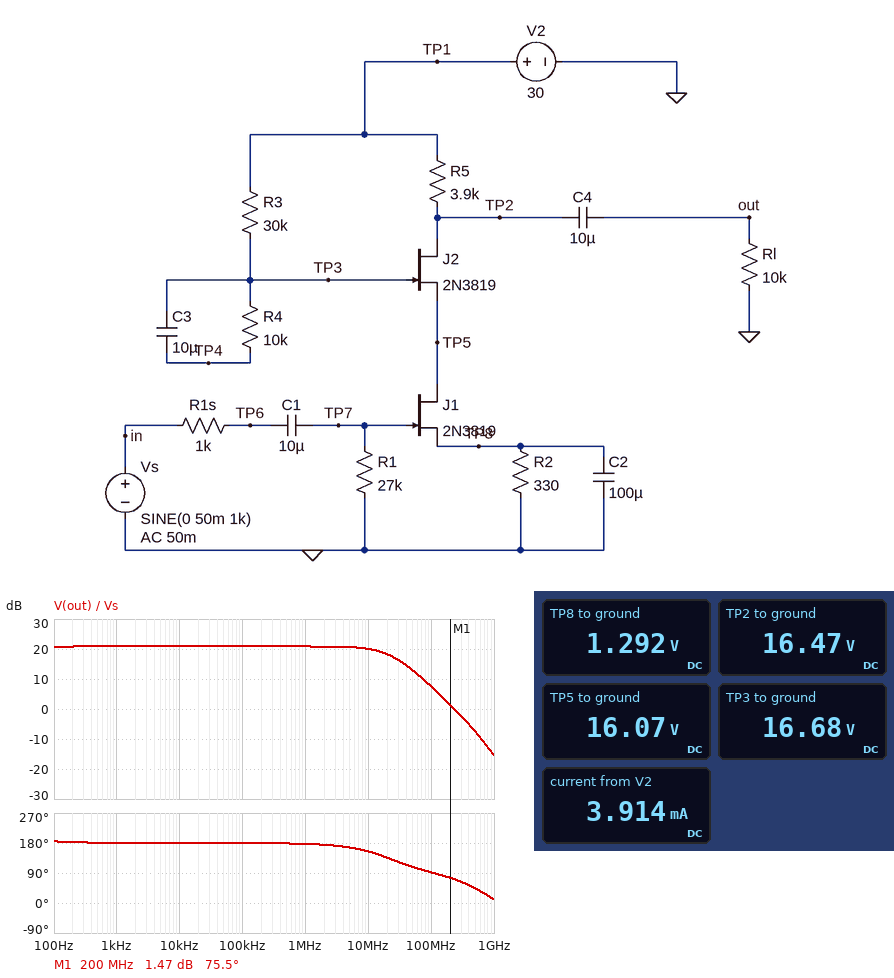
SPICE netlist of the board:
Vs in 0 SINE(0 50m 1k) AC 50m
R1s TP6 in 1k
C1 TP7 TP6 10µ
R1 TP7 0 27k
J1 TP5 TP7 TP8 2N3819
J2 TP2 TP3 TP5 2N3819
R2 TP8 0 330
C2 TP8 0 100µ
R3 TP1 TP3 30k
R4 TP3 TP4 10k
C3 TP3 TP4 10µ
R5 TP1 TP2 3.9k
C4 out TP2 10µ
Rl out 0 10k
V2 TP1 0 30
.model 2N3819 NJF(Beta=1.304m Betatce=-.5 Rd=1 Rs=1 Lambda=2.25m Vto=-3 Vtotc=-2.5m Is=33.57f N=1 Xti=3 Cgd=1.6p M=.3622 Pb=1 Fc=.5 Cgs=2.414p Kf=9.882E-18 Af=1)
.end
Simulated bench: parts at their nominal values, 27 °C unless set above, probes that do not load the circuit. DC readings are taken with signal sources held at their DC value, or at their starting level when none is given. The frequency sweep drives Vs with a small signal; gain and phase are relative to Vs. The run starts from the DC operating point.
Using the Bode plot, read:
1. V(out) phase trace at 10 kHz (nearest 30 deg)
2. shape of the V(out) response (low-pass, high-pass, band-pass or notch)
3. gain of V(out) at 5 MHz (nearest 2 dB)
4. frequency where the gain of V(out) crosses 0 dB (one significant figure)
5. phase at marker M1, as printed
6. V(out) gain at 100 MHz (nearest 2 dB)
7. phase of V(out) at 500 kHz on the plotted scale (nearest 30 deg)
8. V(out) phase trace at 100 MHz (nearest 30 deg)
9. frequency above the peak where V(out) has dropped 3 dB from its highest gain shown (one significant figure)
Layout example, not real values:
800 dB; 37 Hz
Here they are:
180 deg; low-pass; 20 dB; 200 MHz; 75.5 deg; 8 dB; 180 deg; 90 deg; 20 MHz
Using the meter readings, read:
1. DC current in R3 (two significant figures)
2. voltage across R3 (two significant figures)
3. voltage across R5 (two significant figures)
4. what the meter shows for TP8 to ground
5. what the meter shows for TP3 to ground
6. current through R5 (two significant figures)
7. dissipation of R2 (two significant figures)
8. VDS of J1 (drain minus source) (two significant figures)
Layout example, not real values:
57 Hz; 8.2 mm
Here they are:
440 µA; 13 V; 14 V; 1.292 V; 16.68 V; 3.5 mA; 5.1 mW; 15 V
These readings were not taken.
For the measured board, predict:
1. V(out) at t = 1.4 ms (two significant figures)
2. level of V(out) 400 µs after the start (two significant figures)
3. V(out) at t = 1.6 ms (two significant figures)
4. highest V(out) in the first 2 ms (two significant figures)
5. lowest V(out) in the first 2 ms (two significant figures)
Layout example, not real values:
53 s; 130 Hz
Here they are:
-320 mV; -320 mV; 330 mV; 550 mV; -550 mV
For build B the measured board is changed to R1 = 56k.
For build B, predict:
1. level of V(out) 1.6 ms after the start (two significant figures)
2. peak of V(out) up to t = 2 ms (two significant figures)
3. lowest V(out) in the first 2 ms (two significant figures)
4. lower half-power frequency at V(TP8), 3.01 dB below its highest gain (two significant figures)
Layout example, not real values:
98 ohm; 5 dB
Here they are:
340 mV; 560 mV; -560 mV; 270 mHz
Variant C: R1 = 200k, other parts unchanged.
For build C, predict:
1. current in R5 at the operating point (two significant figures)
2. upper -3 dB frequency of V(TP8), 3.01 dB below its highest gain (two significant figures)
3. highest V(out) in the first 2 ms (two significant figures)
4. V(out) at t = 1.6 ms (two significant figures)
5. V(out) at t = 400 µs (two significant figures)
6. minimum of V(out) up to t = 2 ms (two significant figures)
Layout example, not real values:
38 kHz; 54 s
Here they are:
3.5 mA; 12 Hz; 570 mV; 340 mV; -330 mV; -570 mV
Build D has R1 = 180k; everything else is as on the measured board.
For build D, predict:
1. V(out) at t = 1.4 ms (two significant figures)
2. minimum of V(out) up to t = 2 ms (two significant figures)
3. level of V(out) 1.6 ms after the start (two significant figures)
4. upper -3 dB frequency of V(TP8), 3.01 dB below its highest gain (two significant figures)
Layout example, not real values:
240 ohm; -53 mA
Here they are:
-330 mV; -570 mV; 340 mV; 12 Hz
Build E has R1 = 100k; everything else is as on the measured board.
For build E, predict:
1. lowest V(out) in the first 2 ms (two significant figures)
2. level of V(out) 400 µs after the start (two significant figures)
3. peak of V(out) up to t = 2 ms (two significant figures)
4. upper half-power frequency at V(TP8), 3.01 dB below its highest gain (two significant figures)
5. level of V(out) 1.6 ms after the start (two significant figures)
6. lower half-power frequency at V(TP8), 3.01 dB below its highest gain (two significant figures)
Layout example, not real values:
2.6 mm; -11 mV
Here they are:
-570 mV; -330 mV; 560 mV; 12 Hz; 340 mV; 150 mHz
